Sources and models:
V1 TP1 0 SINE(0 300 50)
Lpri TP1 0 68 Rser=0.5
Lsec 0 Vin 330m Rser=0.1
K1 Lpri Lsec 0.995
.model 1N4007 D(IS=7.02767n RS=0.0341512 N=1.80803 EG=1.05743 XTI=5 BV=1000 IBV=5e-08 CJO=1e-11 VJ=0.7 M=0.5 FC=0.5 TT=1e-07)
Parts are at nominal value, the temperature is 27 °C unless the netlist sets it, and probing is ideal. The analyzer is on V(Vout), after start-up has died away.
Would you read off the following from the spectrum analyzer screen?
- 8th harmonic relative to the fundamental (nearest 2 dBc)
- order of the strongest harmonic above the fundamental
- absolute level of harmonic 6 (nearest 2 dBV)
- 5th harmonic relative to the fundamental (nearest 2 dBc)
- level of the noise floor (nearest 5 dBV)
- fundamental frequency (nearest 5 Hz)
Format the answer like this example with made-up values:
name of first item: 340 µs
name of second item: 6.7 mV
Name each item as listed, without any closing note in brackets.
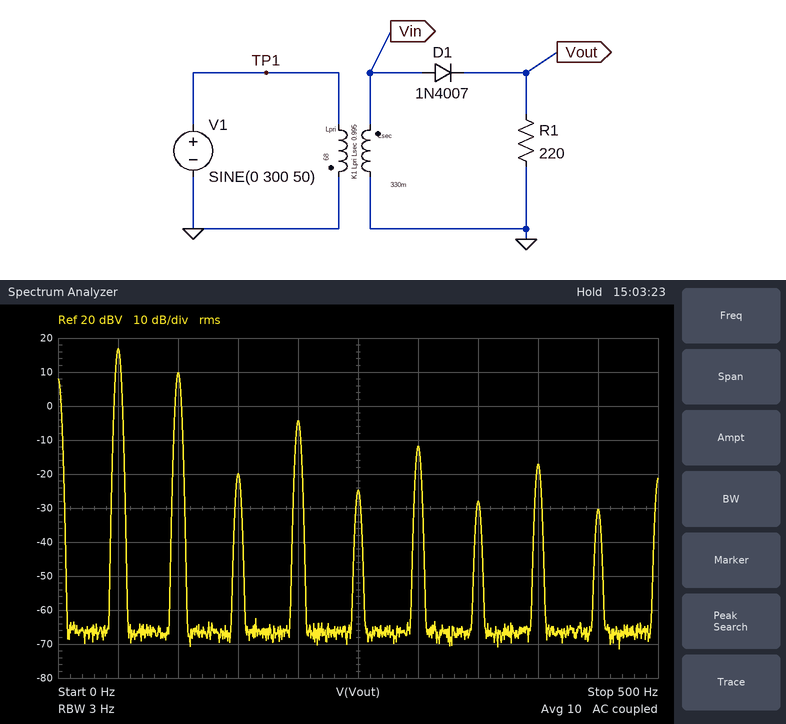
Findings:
8th harmonic relative to the fundamental: -34 dBc
order of the strongest harmonic above the fundamental: 2
absolute level of harmonic 6: -12 dBV
5th harmonic relative to the fundamental: -42 dBc
level of the noise floor: -65 dBV
fundamental frequency: 50 Hz
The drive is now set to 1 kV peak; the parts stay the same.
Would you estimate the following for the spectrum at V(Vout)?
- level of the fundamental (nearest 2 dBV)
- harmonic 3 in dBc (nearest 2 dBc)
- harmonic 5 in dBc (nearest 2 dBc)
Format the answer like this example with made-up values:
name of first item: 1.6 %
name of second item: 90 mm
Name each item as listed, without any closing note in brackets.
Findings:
level of the fundamental: 28 dBV
harmonic 3 in dBc: -46 dBc
harmonic 5 in dBc: -52 dBc
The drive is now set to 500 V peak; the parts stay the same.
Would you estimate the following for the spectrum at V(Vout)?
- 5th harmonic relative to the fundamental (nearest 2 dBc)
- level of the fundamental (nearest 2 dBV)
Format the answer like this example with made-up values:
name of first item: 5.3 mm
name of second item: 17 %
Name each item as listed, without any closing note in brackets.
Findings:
5th harmonic relative to the fundamental: -46 dBc
level of the fundamental: 22 dBV
